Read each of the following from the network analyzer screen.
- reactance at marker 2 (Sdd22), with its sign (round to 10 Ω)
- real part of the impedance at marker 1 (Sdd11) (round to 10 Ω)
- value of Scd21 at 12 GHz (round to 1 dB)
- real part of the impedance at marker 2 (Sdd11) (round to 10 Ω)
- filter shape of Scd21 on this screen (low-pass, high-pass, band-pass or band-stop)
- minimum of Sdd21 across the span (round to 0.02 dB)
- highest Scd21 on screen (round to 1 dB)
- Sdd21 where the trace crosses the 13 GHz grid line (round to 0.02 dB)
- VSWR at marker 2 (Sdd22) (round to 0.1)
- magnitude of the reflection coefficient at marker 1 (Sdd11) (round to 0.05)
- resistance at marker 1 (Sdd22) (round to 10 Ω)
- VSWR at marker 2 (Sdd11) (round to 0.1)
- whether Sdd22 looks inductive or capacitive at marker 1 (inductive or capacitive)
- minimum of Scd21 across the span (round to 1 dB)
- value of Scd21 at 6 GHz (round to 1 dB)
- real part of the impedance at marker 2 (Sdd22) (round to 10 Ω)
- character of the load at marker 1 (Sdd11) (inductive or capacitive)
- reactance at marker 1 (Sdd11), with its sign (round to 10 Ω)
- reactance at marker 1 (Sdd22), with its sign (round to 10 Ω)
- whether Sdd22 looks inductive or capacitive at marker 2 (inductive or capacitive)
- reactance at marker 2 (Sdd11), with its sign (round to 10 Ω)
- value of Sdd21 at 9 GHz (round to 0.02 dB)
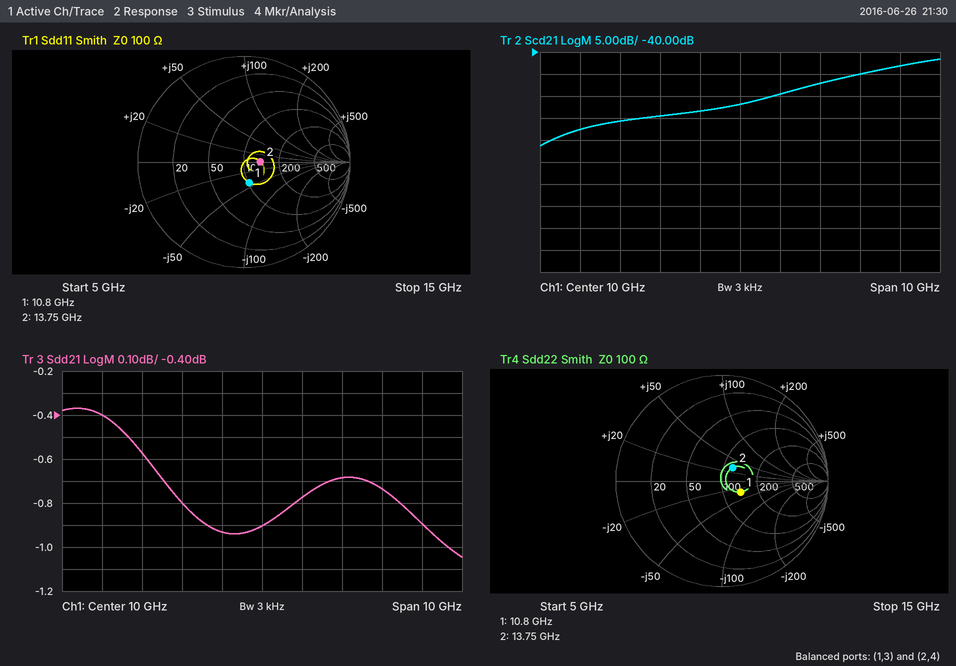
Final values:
+30 Ω
100 Ω
-47 dB
140 Ω
high-pass
-1.04 dB
-42 dB
-0.74 dB
1.4
0.20
140 Ω
1.4
capacitive
-61 dB
-58 dB
120 Ω
capacitive
-40 Ω
-30 Ω
inductive
0 Ω
-0.94 dB
